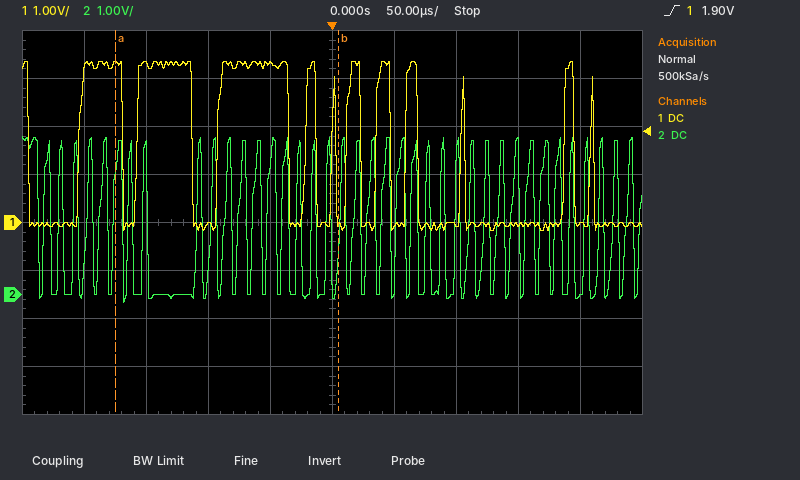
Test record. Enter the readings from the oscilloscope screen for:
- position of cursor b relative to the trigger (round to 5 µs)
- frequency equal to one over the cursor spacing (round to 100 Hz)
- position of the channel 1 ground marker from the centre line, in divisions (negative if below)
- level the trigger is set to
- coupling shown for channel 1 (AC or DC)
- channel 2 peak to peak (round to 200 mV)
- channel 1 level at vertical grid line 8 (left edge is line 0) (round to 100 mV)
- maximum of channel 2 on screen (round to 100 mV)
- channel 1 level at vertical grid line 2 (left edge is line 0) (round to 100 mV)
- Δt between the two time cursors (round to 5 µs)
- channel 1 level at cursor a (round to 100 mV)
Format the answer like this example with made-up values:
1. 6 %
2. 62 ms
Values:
1. +5 µs
2. 5.6 kHz
3. 0.0 div
4. 1.90 V
5. DC
6. 3.4 V
7. 0.0 V
8. 3.3 V
9. 3.3 V
10. 180 µs
11. 3.3 V
